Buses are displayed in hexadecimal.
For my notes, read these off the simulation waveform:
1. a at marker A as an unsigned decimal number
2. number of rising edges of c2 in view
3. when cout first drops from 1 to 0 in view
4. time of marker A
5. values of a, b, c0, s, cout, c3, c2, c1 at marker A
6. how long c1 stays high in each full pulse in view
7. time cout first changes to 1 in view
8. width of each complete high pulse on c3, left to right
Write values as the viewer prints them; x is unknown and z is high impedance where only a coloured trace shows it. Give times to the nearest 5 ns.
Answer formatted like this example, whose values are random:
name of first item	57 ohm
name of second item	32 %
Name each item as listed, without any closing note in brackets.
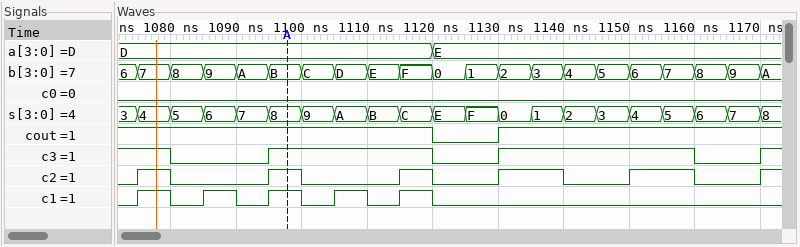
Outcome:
a at marker A as an unsigned decimal number	13
number of rising edges of c2 in view	6
when cout first drops from 1 to 0 in view	1120 ns
time of marker A	1100 ns
values of a, b, c0, s, cout, c3, c2, c1 at marker A	a=D, b=B, c0=0, s=8, cout=1, c3=1, c2=1, c1=1
how long c1 stays high in each full pulse in view	5 ns, 5 ns, 5 ns, 5 ns, 5 ns
time cout first changes to 1 in view	1130 ns
width of each complete high pulse on c3, left to right	25 ns, 30 ns
